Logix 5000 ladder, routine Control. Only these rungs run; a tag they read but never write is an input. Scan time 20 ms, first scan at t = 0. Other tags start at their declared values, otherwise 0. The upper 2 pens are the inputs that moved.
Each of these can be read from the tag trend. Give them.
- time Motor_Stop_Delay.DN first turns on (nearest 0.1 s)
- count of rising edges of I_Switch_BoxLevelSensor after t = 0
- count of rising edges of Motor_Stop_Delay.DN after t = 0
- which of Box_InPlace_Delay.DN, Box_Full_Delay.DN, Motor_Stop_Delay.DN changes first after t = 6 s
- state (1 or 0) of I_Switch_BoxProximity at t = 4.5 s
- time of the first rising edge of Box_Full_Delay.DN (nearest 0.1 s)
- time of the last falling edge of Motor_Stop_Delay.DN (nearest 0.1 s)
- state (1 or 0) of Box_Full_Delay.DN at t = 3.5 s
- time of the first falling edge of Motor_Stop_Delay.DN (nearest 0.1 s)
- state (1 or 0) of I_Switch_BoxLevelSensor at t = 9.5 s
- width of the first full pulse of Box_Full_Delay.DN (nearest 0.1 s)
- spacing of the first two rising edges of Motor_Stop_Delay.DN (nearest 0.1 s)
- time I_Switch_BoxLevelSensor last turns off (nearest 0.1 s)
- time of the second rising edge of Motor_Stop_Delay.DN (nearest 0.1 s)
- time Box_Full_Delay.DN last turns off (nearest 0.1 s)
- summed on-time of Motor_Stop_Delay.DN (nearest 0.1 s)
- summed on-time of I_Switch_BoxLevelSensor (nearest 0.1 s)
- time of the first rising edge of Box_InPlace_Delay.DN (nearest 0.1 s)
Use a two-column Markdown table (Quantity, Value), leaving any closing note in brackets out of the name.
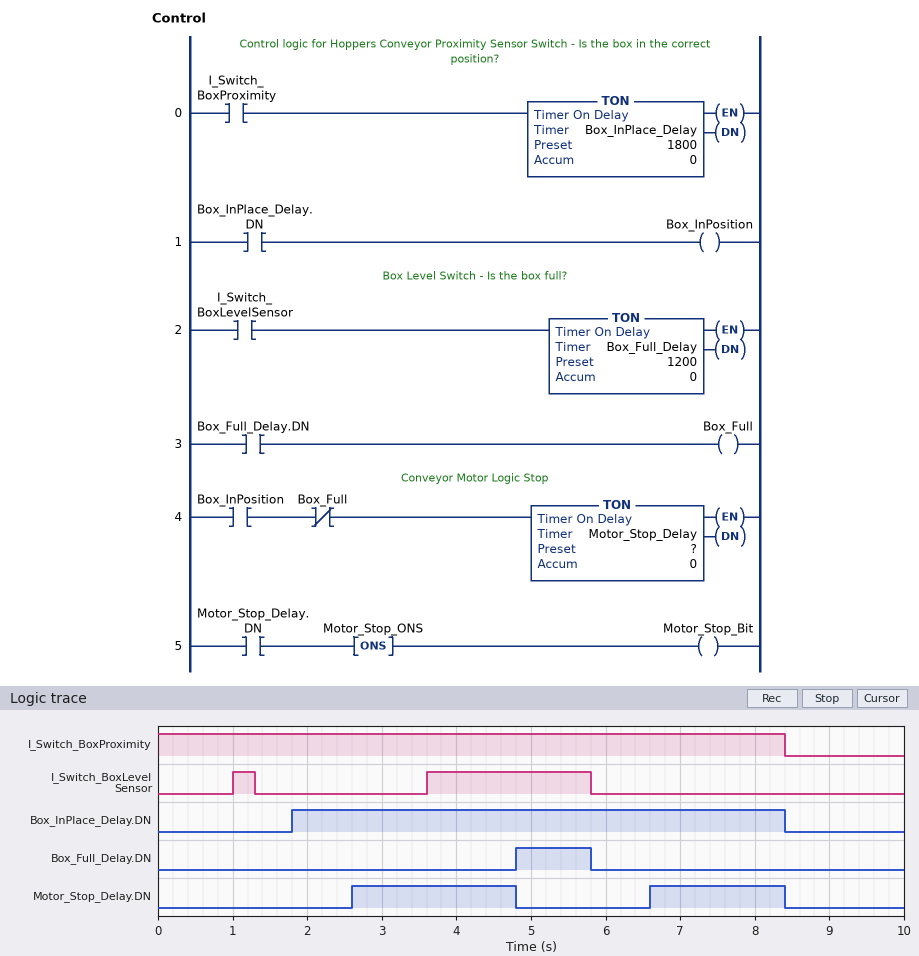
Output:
| Quantity | Value |
|---|---|
| time Motor_Stop_Delay.DN first turns on | 2.6 s |
| count of rising edges of I_Switch_BoxLevelSensor after t = 0 | 2 |
| count of rising edges of Motor_Stop_Delay.DN after t = 0 | 2 |
| which of Box_InPlace_Delay.DN, Box_Full_Delay.DN, Motor_Stop_Delay.DN changes first after t = 6 s | Motor_Stop_Delay.DN |
| state (1 or 0) of I_Switch_BoxProximity at t = 4.5 s | 1 |
| time of the first rising edge of Box_Full_Delay.DN | 4.8 s |
| time of the last falling edge of Motor_Stop_Delay.DN | 8.4 s |
| state (1 or 0) of Box_Full_Delay.DN at t = 3.5 s | 0 |
| time of the first falling edge of Motor_Stop_Delay.DN | 4.8 s |
| state (1 or 0) of I_Switch_BoxLevelSensor at t = 9.5 s | 0 |
| width of the first full pulse of Box_Full_Delay.DN | 1.0 s |
| spacing of the first two rising edges of Motor_Stop_Delay.DN | 4.0 s |
| time I_Switch_BoxLevelSensor last turns off | 5.8 s |
| time of the second rising edge of Motor_Stop_Delay.DN | 6.6 s |
| time Box_Full_Delay.DN last turns off | 5.8 s |
| summed on-time of Motor_Stop_Delay.DN | 4.0 s |
| summed on-time of I_Switch_BoxLevelSensor | 2.5 s |
| time of the first rising edge of Box_InPlace_Delay.DN | 1.8 s |
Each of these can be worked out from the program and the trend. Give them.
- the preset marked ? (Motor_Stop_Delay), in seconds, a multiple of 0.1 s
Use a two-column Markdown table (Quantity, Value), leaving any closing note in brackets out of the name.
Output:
| Quantity | Value |
|---|---|
| the preset marked ? (Motor_Stop_Delay), in seconds, a multiple of 0.1 s | 0.8 s |
